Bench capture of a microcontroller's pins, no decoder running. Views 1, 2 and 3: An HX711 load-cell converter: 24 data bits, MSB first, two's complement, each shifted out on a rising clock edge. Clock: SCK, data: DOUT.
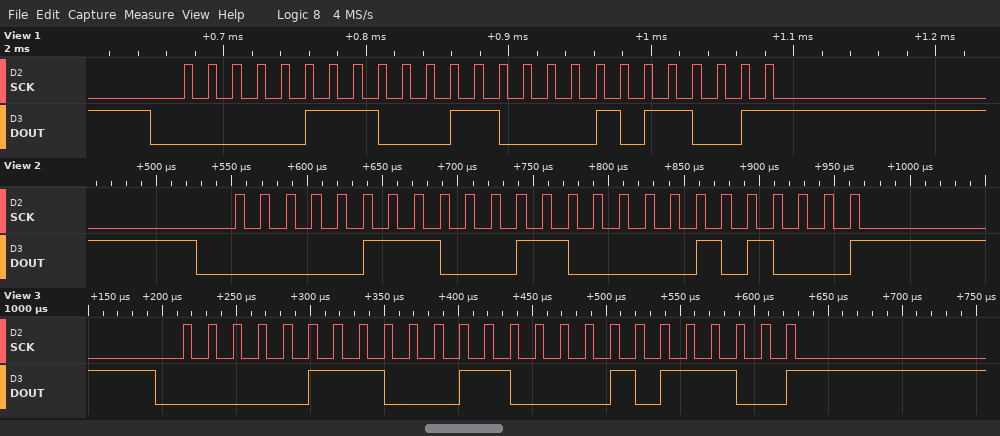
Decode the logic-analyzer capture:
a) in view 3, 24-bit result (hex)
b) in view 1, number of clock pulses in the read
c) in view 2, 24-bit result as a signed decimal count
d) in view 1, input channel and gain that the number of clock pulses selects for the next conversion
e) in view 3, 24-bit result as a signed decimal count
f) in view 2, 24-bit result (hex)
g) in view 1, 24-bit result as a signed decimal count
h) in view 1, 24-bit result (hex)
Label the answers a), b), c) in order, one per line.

a) 0x07185C
b) 25
c) 464936
d) channel A, gain 128
e) 464988
f) 0x071828
g) 464985
h) 0x071859
